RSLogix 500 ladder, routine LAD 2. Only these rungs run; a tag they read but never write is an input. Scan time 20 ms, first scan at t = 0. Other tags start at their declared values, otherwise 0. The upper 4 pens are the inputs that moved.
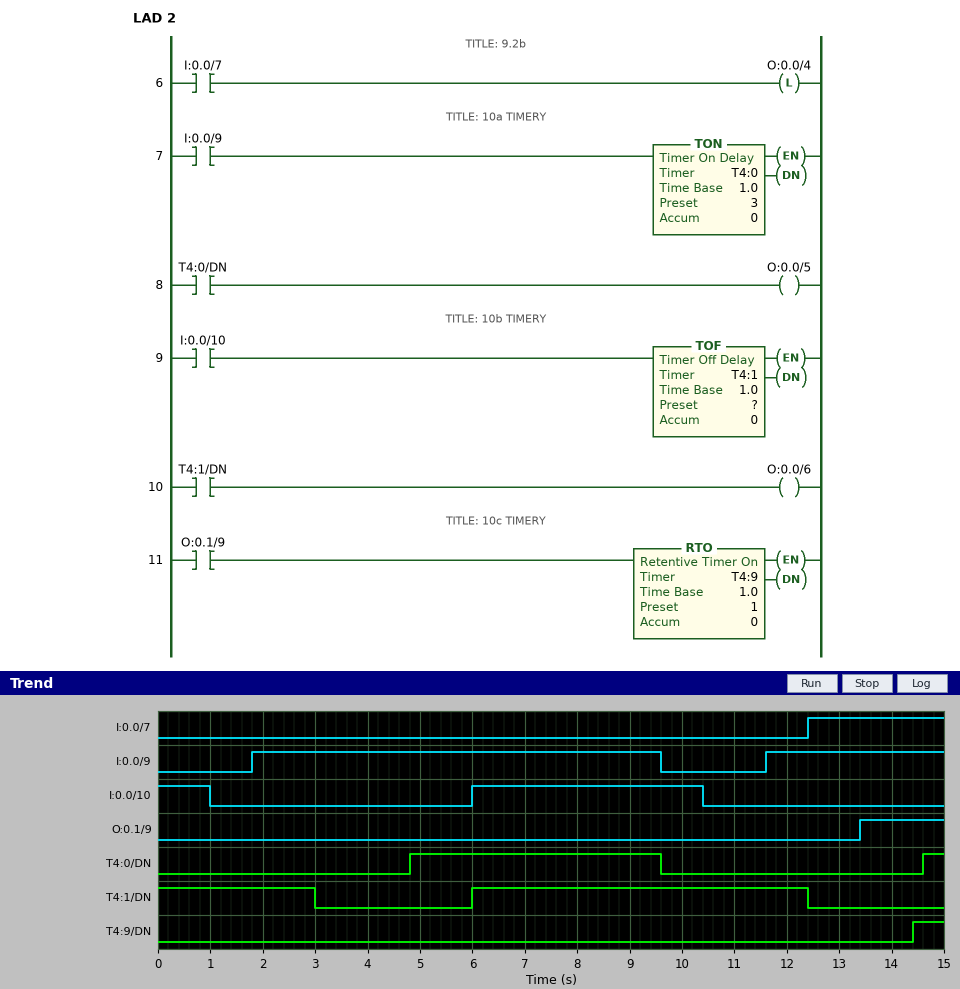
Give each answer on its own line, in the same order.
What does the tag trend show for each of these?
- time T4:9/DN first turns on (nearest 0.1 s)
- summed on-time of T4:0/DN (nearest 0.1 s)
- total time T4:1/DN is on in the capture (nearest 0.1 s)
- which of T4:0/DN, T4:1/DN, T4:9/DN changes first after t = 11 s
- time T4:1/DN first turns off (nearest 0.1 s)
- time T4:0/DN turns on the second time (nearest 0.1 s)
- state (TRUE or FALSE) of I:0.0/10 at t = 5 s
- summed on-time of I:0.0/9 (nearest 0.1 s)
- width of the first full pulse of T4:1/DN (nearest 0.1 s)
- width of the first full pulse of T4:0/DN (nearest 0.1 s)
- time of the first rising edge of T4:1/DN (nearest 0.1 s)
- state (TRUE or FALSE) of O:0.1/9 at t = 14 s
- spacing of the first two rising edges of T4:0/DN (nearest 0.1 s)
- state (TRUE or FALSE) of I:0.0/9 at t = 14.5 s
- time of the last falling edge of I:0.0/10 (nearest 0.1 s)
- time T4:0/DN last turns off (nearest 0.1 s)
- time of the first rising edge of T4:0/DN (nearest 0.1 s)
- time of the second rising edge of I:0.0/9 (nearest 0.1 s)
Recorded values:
14.4 s
5.2 s
9.4 s
T4:1/DN
3.0 s
14.6 s
FALSE
11.2 s
6.4 s
4.8 s
6.0 s
TRUE
9.8 s
TRUE
10.4 s
9.6 s
4.8 s
11.6 s
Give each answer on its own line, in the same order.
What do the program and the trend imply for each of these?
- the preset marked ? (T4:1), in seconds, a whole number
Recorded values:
2 s
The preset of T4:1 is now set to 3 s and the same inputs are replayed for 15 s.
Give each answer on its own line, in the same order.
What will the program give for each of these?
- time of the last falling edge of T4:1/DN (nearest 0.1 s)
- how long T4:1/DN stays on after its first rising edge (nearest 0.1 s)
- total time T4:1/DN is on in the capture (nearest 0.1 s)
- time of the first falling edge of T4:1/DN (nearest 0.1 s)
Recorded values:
13.4 s
7.4 s
11.4 s
4.0 s
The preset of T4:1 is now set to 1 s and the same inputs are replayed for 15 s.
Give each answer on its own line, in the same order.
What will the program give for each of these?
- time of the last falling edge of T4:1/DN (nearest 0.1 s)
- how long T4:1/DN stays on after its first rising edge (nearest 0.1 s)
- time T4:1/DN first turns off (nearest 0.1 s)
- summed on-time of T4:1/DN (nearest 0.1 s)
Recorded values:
11.4 s
5.4 s
2.0 s
7.4 s
